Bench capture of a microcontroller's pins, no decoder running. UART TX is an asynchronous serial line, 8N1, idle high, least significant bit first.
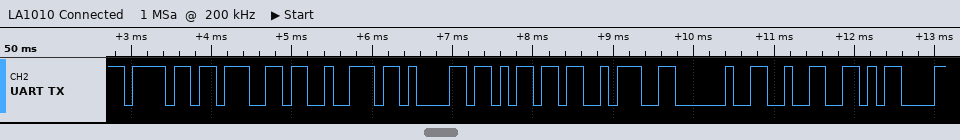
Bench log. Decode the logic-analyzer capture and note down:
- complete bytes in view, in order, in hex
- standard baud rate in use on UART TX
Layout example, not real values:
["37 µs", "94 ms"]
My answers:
["0x6F 0x67 0x72 0x61 0x6D 0x3A 0x20 0x32 0x0D", "9600 baud"]
